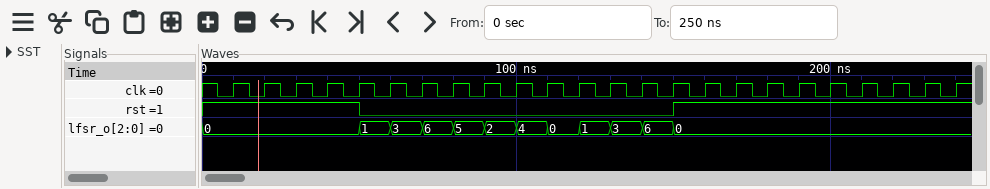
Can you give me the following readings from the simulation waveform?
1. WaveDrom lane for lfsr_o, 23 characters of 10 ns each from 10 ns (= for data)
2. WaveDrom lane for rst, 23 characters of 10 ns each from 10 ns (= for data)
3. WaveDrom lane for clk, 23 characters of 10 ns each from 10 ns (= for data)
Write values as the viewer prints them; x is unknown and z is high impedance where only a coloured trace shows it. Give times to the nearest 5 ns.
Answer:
{name: 'lfsr_o', wave: '=...===========........', data: '0 1 3 6 5 2 4 0 1 3 6 0'}
{name: 'rst', wave: '1...0.........1........'}
{name: 'clk', wave: 'p......................'}
